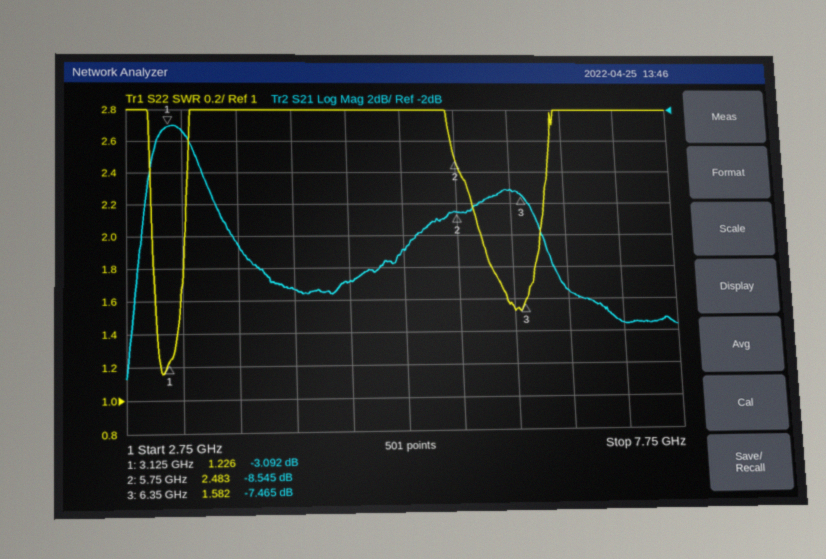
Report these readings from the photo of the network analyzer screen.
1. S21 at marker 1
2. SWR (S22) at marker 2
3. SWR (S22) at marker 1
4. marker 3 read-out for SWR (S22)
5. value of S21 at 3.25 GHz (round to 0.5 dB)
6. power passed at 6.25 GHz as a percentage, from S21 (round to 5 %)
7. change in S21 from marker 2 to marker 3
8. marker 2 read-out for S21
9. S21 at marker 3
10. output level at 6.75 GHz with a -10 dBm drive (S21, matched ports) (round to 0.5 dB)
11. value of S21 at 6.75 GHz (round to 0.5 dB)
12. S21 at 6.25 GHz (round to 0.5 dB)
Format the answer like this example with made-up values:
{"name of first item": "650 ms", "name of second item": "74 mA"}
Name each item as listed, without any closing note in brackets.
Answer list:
{"S21 at marker 1": "-3.092 dB", "SWR (S22) at marker 2": "2.483", "SWR (S22) at marker 1": "1.226", "marker 3 read-out for SWR": "1.582", "value of S21 at 3.25 GHz": "-3.5 dB", "power passed at 6.25 GHz as a percentage, from S21": "20 %", "change in S21 from marker 2 to marker 3": "1.080 dB", "marker 2 read-out for S21": "-8.545 dB", "S21 at marker 3": "-7.465 dB", "output level at 6.75 GHz with a -10 dBm drive (S21, matched ports)": "-23.5 dBm", "value of S21 at 6.75 GHz": "-13.5 dB", "S21 at 6.25 GHz": "-7.0 dB"}
